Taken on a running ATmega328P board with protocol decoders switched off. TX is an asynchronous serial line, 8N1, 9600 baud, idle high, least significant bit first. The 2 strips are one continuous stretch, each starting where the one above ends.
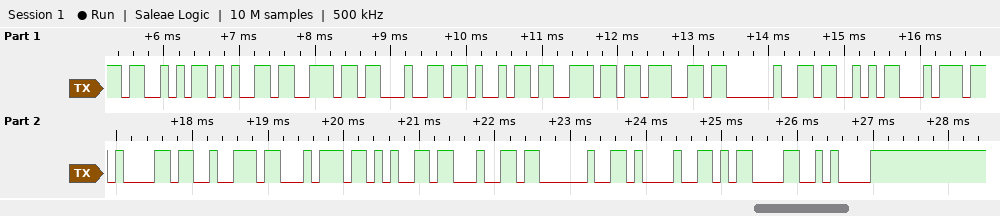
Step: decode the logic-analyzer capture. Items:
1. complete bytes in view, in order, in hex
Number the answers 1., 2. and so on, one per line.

1. 53 65 6E 64 69 6E 67 20 53 74 61 72 74 65 64 20 21 0D 0A
